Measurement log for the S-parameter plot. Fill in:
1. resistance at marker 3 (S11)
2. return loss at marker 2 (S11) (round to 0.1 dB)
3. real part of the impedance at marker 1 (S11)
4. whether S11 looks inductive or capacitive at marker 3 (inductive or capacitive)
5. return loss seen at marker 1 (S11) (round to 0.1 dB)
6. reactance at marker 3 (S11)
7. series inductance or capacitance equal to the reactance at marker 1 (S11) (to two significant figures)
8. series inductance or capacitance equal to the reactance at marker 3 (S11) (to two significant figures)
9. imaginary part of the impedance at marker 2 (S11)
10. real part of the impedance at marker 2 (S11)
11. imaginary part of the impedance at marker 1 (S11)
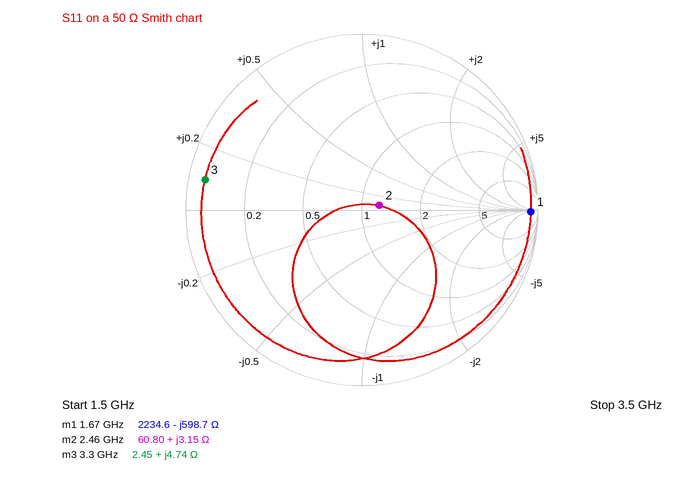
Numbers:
2.45 Ω
19.9 dB
2234.6 Ω
inductive
0.4 dB
+4.74 Ω
160 fF
230 pH
+3.15 Ω
60.80 Ω
-598.7 Ω
